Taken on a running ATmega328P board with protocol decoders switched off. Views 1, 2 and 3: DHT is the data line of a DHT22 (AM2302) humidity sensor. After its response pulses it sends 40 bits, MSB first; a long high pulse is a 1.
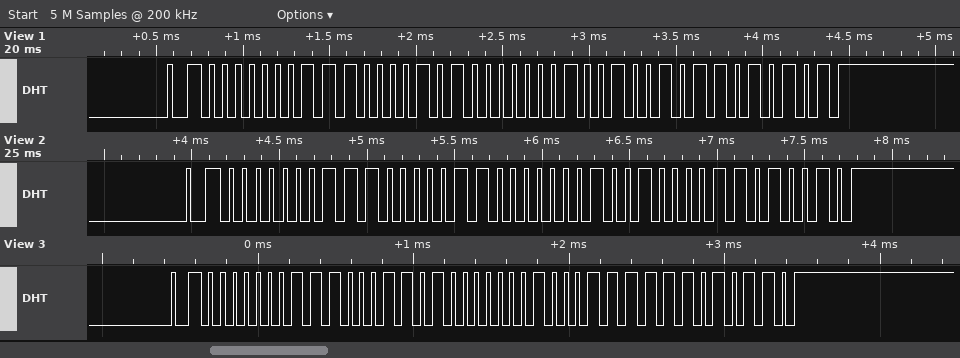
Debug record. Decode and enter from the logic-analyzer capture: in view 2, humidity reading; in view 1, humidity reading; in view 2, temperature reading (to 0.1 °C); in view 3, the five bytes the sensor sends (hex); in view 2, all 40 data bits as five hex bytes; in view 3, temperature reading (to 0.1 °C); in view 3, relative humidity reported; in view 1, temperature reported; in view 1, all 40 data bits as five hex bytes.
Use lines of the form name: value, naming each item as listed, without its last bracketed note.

in view 2, humidity reading: 44.9 %
in view 1, humidity reading: 45.0 %
in view 2, temperature reading: -14.4 °C
in view 3, the five bytes the sensor sends: 01 C6 80 8F D6
in view 2, all 40 data bits as five hex bytes: 01 C1 80 90 D2
in view 3, temperature reading: -14.3 °C
in view 3, relative humidity reported: 45.4 %
in view 1, temperature reported: -14.6 °C
in view 1, all 40 data bits as five hex bytes: 01 C2 80 92 D5
